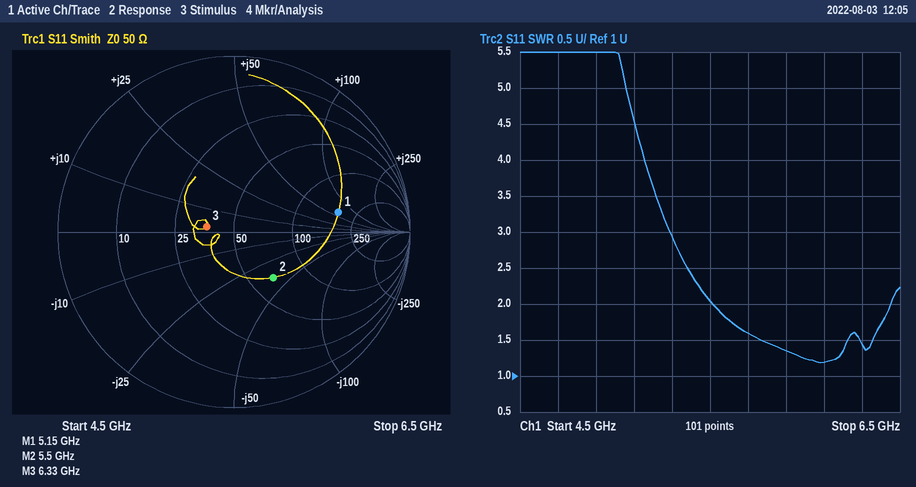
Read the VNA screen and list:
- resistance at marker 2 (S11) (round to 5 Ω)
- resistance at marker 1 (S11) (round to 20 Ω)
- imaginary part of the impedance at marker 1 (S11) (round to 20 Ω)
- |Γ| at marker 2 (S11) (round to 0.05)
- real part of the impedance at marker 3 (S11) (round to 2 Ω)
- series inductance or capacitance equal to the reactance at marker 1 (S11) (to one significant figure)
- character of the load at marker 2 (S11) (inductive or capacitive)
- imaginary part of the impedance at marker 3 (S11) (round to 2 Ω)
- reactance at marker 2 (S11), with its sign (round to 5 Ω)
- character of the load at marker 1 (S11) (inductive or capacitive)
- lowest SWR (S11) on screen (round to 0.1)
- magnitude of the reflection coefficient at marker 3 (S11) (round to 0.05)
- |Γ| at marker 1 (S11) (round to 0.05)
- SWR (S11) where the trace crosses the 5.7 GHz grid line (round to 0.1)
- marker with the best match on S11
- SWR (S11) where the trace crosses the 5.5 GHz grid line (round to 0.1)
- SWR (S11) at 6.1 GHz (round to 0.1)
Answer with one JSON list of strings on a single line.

["65 Ω", "180 Ω", "+60 Ω", "0.35", "36 Ω", "2 nH", "capacitive", "+2 Ω", "-40 Ω", "inductive", "1.2", "0.15", "0.60", "1.6", "marker 3", "2.0", "1.2"]
